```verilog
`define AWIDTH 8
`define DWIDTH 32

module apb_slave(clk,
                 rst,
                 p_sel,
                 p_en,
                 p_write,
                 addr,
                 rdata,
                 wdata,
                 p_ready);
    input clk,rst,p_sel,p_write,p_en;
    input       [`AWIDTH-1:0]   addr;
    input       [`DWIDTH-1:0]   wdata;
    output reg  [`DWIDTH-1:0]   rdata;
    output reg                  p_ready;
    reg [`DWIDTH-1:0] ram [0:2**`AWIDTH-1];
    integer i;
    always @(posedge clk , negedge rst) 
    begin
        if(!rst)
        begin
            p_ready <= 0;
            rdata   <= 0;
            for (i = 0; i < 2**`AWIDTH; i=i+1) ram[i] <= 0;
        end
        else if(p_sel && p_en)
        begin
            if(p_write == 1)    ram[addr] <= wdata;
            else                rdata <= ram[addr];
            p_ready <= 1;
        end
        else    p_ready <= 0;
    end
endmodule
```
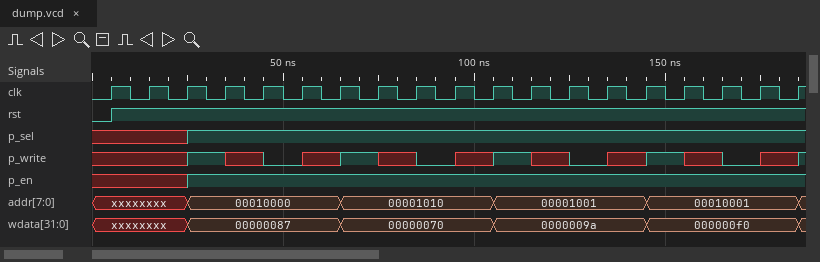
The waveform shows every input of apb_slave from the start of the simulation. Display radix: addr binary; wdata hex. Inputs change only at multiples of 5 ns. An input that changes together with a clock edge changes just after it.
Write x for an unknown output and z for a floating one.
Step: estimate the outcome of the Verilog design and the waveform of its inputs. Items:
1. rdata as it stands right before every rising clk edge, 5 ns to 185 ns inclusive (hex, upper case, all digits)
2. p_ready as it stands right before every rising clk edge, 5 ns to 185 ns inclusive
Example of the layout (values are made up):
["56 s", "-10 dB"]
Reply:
["00000000, 00000000, 00000000, 00000000, 00000000, 00000087, 00000087, 00000087, 00000087, 00000070, 00000070, 00000070, 00000070, 0000009A, 0000009A, 0000009A, 0000009A, 000000F0, 000000F0", "0 0 0 0 1 1 1 1 1 1 1 1 1 1 1 1 1 1 1"]
